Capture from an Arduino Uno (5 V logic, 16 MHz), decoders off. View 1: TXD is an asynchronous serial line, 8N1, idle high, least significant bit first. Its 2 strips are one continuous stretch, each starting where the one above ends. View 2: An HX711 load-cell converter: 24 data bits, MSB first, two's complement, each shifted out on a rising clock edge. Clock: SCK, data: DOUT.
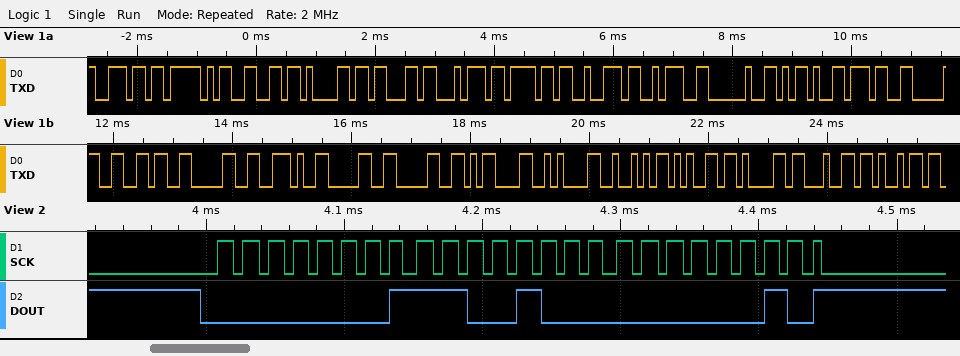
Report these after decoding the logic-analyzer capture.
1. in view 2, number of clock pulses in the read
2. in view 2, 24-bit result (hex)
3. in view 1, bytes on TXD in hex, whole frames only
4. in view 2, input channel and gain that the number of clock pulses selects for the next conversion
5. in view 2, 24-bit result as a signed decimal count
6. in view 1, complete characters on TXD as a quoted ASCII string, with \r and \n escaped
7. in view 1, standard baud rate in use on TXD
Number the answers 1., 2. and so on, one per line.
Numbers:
1. 25
2. 0x01C802
3. 0x6E 0x5F 0x66 0x61 0x63 0x74 0x6F 0x72 0x3A 0x20 0x2D 0x37 0x30 0x36 0x30 0x2E 0x30 0x30 0x0D 0x0A 0x52 0x65 0x61 0x64 0x69
4. channel A, gain 128
5. 116738
6. "n_factor: -7060.00\r\nReadi"
7. 9600 baud
